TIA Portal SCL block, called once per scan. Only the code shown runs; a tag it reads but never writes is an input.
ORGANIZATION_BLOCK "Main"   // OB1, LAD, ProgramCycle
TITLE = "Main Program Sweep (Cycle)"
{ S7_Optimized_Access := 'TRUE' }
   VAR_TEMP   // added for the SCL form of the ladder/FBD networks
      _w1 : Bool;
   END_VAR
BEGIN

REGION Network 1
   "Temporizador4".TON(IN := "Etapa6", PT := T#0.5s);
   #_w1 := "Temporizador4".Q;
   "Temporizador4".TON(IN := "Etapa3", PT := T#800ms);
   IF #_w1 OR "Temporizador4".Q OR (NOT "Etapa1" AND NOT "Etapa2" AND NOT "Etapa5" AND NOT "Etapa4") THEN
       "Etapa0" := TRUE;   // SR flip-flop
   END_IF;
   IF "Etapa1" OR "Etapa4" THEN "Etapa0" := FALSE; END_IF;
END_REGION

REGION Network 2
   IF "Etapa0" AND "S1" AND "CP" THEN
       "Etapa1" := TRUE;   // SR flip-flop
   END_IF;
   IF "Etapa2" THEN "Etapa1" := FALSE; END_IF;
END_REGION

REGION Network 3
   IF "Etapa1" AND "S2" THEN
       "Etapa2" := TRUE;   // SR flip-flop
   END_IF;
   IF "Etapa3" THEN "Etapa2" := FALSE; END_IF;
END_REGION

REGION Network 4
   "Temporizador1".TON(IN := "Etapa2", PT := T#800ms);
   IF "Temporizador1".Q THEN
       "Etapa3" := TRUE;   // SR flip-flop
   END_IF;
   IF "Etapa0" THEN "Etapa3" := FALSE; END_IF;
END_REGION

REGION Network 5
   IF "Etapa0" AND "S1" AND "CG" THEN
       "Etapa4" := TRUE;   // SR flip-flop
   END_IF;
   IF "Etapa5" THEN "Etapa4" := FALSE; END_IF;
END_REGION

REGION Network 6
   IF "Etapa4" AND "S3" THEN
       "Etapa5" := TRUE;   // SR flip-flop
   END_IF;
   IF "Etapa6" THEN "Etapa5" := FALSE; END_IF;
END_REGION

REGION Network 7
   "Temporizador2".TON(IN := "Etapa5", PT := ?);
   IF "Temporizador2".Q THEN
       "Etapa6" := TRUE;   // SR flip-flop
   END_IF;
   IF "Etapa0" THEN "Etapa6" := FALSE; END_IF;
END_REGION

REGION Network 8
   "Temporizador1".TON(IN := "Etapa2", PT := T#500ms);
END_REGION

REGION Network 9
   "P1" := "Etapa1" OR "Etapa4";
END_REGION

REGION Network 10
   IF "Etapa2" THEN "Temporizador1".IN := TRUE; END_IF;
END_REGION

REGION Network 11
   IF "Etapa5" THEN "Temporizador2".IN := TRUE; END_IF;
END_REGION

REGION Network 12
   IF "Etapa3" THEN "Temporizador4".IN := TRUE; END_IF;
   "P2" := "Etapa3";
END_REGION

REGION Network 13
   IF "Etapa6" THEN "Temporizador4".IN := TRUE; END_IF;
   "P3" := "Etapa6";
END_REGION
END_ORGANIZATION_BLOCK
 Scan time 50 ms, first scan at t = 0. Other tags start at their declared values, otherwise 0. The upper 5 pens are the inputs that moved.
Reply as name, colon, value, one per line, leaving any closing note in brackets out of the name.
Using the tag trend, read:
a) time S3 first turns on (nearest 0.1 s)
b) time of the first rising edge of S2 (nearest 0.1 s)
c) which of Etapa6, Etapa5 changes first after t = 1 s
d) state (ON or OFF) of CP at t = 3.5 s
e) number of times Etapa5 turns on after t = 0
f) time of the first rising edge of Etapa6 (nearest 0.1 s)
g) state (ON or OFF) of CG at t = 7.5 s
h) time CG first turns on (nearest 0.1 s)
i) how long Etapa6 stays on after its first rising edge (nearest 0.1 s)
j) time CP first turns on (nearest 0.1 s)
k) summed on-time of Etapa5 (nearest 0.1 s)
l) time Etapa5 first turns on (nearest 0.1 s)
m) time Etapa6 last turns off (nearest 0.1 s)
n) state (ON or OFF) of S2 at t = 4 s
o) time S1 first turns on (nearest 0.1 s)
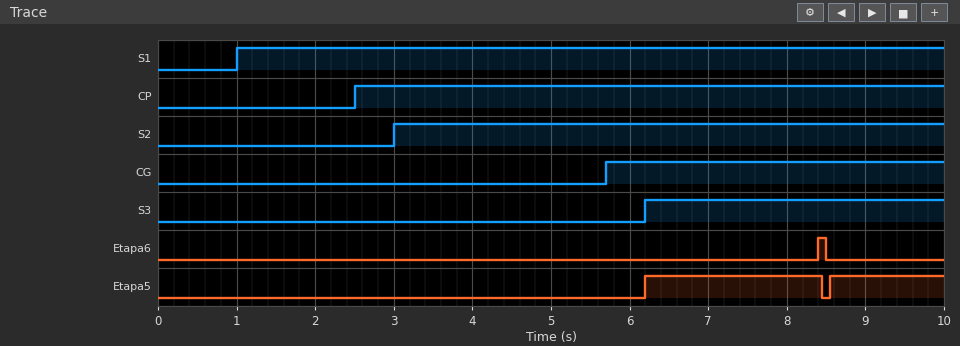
time S3 first turns on: 6.2 s
time of the first rising edge of S2: 3.0 s
which of Etapa6, Etapa5 changes first after t = 1 s: Etapa5
state (ON or OFF) of CP at t = 3.5 s: ON
number of times Etapa5 turns on after t = 0: 2
time of the first rising edge of Etapa6: 8.4 s
state (ON or OFF) of CG at t = 7.5 s: ON
time CG first turns on: 5.7 s
how long Etapa6 stays on after its first rising edge: 0.1 s
time CP first turns on: 2.5 s
summed on-time of Etapa5: 3.7 s
time Etapa5 first turns on: 6.2 s
time Etapa6 last turns off: 8.5 s
state (ON or OFF) of S2 at t = 4 s: ON
time S1 first turns on: 1.0 s
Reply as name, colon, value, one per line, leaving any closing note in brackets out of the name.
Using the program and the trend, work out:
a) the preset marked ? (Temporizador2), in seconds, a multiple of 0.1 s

the preset marked ? (Temporizador2), in seconds, a multiple of 0.1 s: 2.2 s
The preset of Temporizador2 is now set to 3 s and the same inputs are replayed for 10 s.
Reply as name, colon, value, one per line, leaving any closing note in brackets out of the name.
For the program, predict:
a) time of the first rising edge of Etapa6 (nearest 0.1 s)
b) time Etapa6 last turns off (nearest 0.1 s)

time of the first rising edge of Etapa6: 9.2 s
time Etapa6 last turns off: 9.3 s
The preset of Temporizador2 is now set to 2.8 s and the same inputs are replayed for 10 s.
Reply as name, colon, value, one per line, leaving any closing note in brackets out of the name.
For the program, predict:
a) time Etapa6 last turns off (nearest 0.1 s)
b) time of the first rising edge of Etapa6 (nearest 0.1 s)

time Etapa6 last turns off: 9.1 s
time of the first rising edge of Etapa6: 9.0 s
